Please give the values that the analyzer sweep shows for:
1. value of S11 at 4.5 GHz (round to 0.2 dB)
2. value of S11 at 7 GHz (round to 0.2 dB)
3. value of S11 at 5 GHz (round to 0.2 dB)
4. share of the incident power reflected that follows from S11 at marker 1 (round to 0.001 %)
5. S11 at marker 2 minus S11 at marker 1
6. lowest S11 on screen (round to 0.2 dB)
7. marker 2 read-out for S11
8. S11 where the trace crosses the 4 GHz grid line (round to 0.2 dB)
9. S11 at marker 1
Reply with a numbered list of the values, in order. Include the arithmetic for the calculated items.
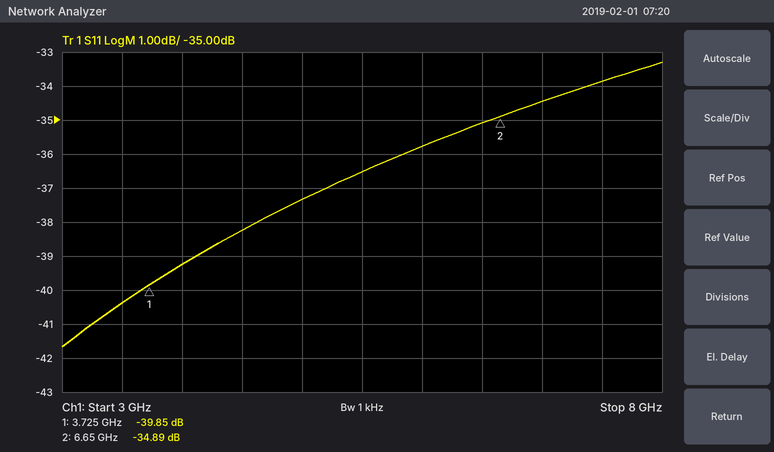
1. -38.2 dB
2. -34.4 dB
3. -37.4 dB
4. 10^(-39.85/10) ≈ 0.010 %
5. -34.89 − (-39.85) = 4.96 dB
6. -41.6 dB
7. -34.89 dB
8. -39.2 dB
9. -39.85 dB
